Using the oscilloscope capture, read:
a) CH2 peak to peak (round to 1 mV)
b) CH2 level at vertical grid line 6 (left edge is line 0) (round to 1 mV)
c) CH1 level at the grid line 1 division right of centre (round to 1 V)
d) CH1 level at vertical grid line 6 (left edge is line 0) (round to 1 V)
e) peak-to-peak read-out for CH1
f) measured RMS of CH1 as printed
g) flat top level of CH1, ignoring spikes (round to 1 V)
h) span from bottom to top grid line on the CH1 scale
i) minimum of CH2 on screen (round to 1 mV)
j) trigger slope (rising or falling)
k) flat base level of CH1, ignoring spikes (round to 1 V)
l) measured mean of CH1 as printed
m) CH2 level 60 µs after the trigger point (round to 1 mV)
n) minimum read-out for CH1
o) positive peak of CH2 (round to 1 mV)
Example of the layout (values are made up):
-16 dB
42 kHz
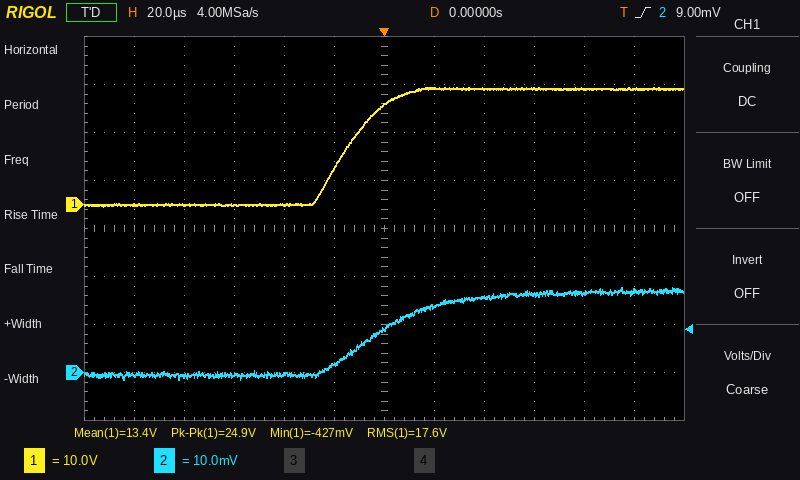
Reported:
19 mV
9 mV
24 V
21 V
24.9 V
17.6 V
24 V
80 V
-1 mV
rising
0 V
13.4 V
16 mV
-427 mV
18 mV
